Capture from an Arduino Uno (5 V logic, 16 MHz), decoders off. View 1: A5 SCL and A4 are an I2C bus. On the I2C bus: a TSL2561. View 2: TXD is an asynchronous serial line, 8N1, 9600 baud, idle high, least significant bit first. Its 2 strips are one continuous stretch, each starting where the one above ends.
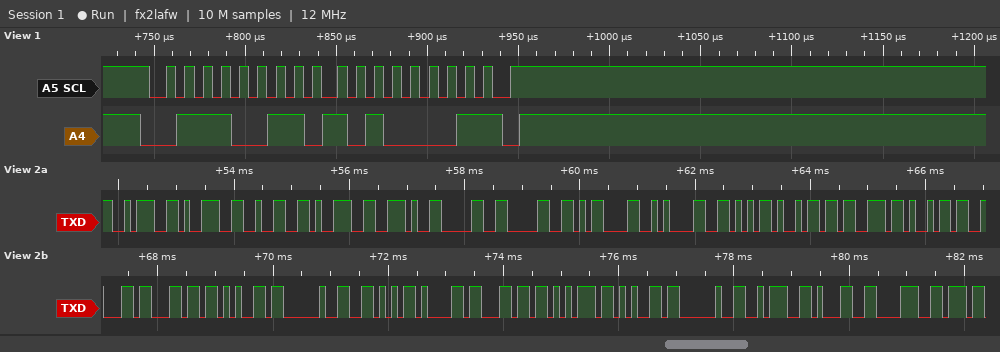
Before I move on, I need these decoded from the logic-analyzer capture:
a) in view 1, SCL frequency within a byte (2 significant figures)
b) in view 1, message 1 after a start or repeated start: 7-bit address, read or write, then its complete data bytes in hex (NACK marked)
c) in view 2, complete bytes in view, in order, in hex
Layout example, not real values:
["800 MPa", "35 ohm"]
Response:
["100 kHz", "0x39 read: A1 NACK", "3A 39 32 39 2E 30 30 0D 0A 56 69 73 69 62 6C 65 20 56 61 6C 75 65 20 3A 31 38"]
